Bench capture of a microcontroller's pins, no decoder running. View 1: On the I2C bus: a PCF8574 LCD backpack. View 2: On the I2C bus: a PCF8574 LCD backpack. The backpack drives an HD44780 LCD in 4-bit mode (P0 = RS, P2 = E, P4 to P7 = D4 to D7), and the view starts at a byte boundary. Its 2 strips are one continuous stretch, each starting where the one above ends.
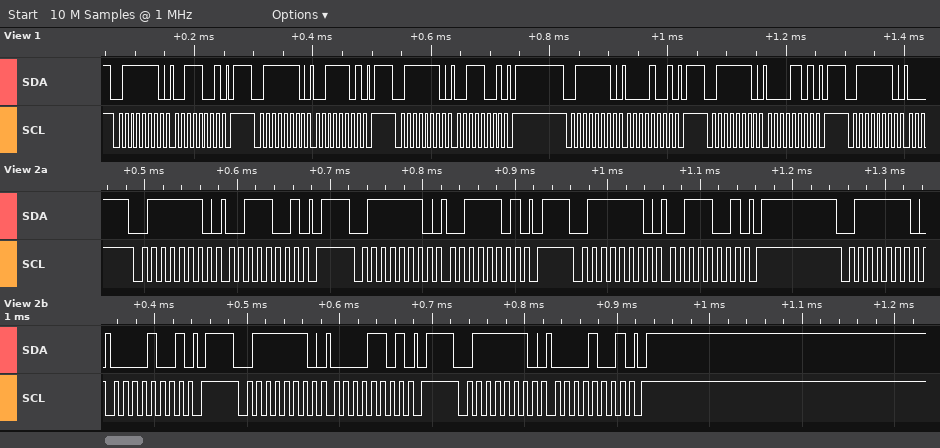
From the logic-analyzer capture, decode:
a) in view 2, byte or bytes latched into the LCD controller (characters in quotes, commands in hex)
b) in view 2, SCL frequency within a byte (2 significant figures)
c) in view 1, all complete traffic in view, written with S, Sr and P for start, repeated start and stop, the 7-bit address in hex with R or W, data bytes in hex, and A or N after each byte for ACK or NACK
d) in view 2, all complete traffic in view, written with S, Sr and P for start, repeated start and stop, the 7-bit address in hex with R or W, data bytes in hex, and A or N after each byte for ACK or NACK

'0'
100 kHz
S 3FW A 39 A P S 3FW A 3D A P S 3FW A 39 A P S 3FW A 09 A P S 3FW A 0D A P S 3FW A
S 3FW A 39 A P S 3FW A 3D A P S 3FW A 39 A P S 3FW A 09 A P S 3FW A 0D A P S 3FW A 09 A P
